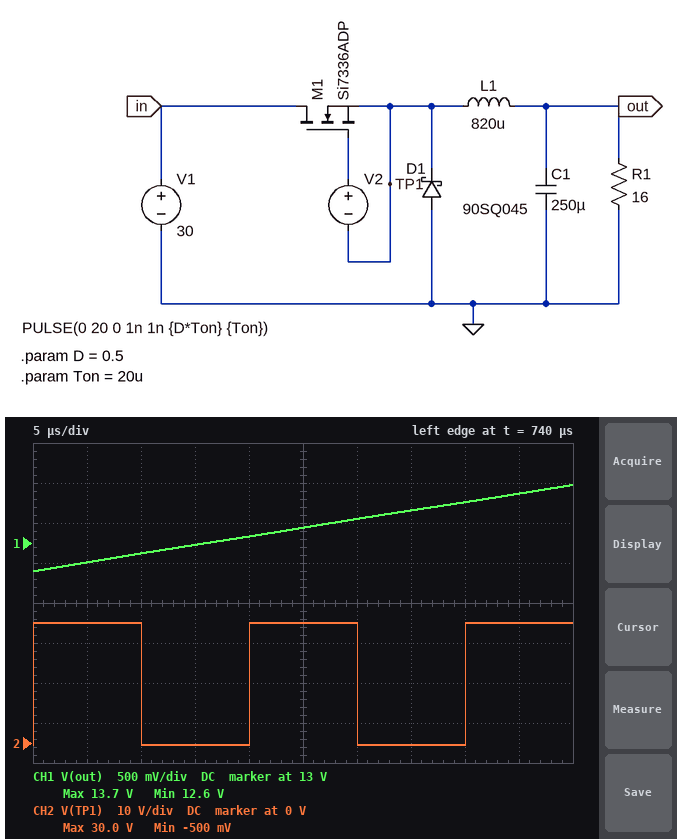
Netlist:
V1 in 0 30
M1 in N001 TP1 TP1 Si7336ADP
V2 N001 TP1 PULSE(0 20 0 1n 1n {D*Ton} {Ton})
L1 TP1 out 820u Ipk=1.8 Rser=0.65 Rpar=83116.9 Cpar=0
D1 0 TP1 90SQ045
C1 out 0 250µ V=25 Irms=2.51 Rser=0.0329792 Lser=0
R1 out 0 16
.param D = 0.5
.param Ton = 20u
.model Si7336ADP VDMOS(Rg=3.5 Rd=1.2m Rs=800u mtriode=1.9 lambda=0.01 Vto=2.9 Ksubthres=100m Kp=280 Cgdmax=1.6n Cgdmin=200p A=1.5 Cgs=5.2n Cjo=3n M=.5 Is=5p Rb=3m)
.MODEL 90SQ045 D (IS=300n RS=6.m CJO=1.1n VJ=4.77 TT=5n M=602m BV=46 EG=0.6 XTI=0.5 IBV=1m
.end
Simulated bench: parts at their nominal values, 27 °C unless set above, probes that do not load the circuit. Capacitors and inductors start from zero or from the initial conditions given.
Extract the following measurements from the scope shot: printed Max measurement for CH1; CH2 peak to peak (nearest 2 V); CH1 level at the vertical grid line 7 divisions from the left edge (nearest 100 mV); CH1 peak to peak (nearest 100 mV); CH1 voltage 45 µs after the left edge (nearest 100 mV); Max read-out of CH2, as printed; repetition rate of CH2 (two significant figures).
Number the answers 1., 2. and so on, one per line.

1. 13.7 V
2. 30 V
3. 13.4 V
4. 1.1 V
5. 13.6 V
6. 30.0 V
7. 50 kHz
